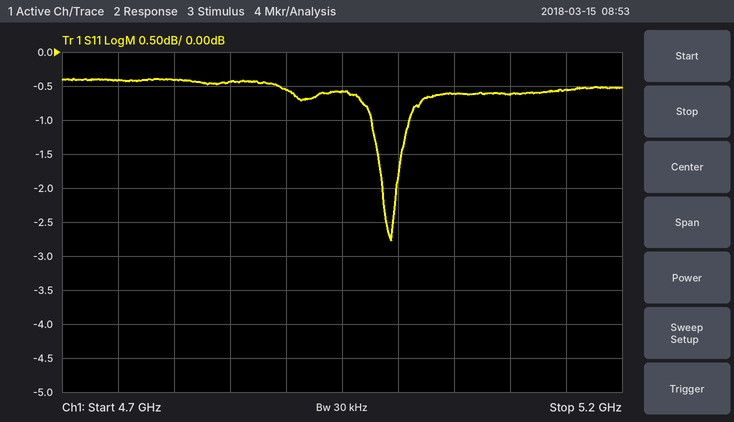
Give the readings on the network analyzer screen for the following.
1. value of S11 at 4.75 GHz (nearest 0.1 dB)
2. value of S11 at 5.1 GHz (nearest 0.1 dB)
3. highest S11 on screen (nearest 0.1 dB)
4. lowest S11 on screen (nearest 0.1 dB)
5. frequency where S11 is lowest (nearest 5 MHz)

-0.4 dB
-0.6 dB
-0.4 dB
-2.8 dB
4.995 GHz
